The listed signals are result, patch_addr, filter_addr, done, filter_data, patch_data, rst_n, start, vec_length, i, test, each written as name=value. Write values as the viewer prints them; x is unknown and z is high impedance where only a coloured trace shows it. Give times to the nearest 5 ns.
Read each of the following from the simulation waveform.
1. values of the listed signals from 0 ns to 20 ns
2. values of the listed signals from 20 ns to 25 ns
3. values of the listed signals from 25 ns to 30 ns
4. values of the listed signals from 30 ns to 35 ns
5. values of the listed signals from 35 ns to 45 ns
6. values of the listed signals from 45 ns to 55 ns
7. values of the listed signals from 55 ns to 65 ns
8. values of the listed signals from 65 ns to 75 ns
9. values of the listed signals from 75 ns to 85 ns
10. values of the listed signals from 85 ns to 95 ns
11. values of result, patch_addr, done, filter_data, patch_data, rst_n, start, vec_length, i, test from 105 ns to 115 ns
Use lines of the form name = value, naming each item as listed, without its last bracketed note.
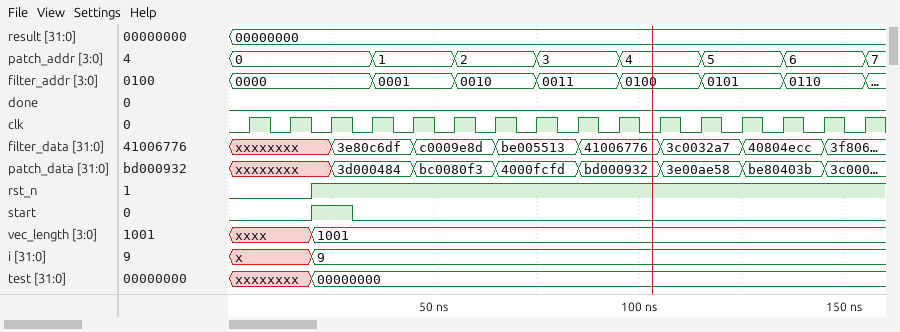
values of the listed signals from 0 ns to 20 ns = result=00000000, patch_addr=0, filter_addr=0000, done=0, filter_data=xxxxxxxx, patch_data=xxxxxxxx, rst_n=0, start=0, vec_length=xxxx, i=x, test=xxxxxxxx
values of the listed signals from 20 ns to 25 ns = result=00000000, patch_addr=0, filter_addr=0000, done=0, filter_data=xxxxxxxx, patch_data=xxxxxxxx, rst_n=1, start=1, vec_length=1001, i=9, test=00000000
values of the listed signals from 25 ns to 30 ns = result=00000000, patch_addr=0, filter_addr=0000, done=0, filter_data=3e80c6df, patch_data=3d000484, rst_n=1, start=1, vec_length=1001, i=9, test=00000000
values of the listed signals from 30 ns to 35 ns = result=00000000, patch_addr=0, filter_addr=0000, done=0, filter_data=3e80c6df, patch_data=3d000484, rst_n=1, start=0, vec_length=1001, i=9, test=00000000
values of the listed signals from 35 ns to 45 ns = result=00000000, patch_addr=1, filter_addr=0001, done=0, filter_data=3e80c6df, patch_data=3d000484, rst_n=1, start=0, vec_length=1001, i=9, test=00000000
values of the listed signals from 45 ns to 55 ns = result=00000000, patch_addr=1, filter_addr=0001, done=0, filter_data=c0009e8d, patch_data=bc0080f3, rst_n=1, start=0, vec_length=1001, i=9, test=00000000
values of the listed signals from 55 ns to 65 ns = result=00000000, patch_addr=2, filter_addr=0010, done=0, filter_data=c0009e8d, patch_data=bc0080f3, rst_n=1, start=0, vec_length=1001, i=9, test=00000000
values of the listed signals from 65 ns to 75 ns = result=00000000, patch_addr=2, filter_addr=0010, done=0, filter_data=be005513, patch_data=4000fcfd, rst_n=1, start=0, vec_length=1001, i=9, test=00000000
values of the listed signals from 75 ns to 85 ns = result=00000000, patch_addr=3, filter_addr=0011, done=0, filter_data=be005513, patch_data=4000fcfd, rst_n=1, start=0, vec_length=1001, i=9, test=00000000
values of the listed signals from 85 ns to 95 ns = result=00000000, patch_addr=3, filter_addr=0011, done=0, filter_data=41006776, patch_data=bd000932, rst_n=1, start=0, vec_length=1001, i=9, test=00000000
values of result, patch_addr, done, filter_data, patch_data, rst_n, start, vec_length, i, test from 105 ns to 115 ns = result=00000000, patch_addr=4, done=0, filter_data=3c0032a7, patch_data=3e00ae58, rst_n=1, start=0, vec_length=1001, i=9, test=00000000
